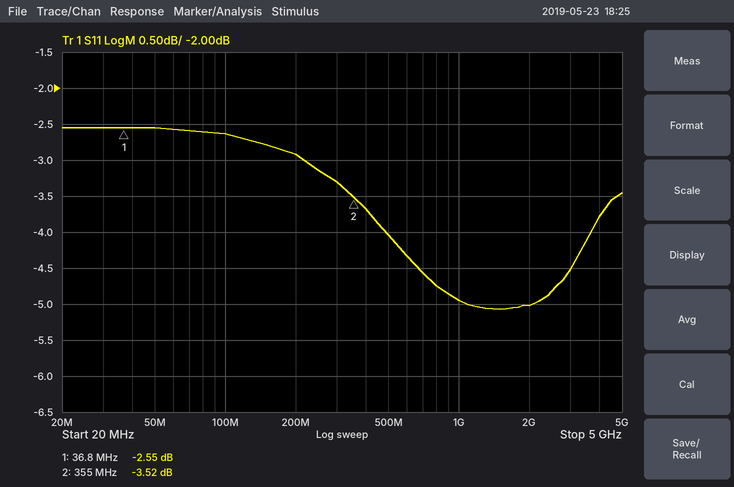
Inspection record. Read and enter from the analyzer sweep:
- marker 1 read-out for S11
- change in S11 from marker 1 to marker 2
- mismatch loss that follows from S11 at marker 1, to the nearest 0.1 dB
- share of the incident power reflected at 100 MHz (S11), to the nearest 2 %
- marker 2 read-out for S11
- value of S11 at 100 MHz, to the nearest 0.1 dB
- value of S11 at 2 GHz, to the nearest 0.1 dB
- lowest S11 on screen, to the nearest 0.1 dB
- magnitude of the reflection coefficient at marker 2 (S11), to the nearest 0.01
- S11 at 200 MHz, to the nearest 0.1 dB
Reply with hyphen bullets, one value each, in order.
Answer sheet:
- -2.55 dB
- -0.97 dB
- 3.5 dB
- 54 %
- -3.52 dB
- -2.6 dB
- -5.0 dB
- -5.1 dB
- 0.67
- -2.9 dB
